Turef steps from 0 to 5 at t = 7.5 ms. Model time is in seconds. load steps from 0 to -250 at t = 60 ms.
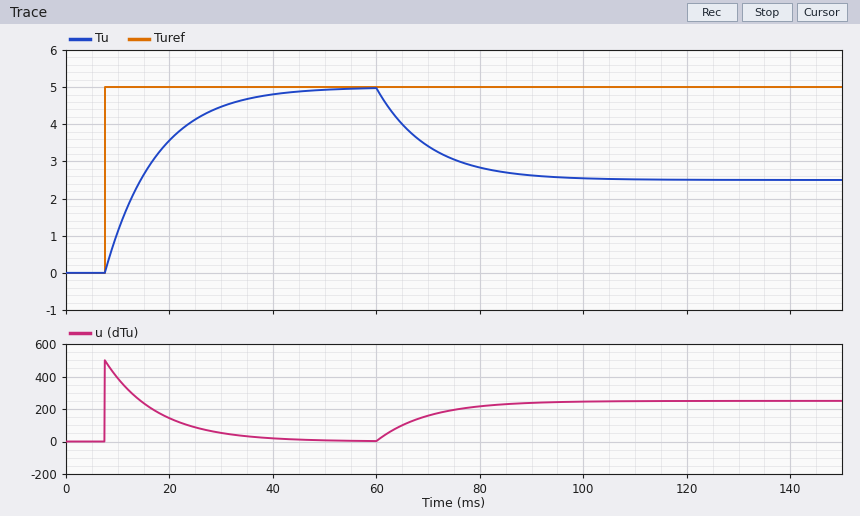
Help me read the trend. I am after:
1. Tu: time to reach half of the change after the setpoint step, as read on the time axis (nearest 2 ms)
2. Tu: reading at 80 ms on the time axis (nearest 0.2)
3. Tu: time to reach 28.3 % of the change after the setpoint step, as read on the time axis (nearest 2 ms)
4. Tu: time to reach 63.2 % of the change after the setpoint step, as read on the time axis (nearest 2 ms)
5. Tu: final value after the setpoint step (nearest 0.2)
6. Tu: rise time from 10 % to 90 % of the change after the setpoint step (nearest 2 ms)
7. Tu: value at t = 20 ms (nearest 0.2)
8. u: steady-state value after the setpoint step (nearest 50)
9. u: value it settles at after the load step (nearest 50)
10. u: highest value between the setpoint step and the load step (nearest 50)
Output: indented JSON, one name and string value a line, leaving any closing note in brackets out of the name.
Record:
{
  "Tu: time to reach half of the change after the setpoint step, as read on the time axis": "14 ms",
  "Tu: reading at 80 ms on the time axis": "2.8",
  "Tu: time to reach 28.3 % of the change after the setpoint step, as read on the time axis": "10 ms",
  "Tu: time to reach 63.2 % of the change after the setpoint step, as read on the time axis": "18 ms",
  "Tu: final value after the setpoint step": "5.0",
  "Tu: rise time from 10 % to 90 % of the change after the setpoint step": "22 ms",
  "Tu: value at t = 20 ms": "3.6",
  "u: steady-state value after the setpoint step": "0",
  "u: value it settles at after the load step": "250",
  "u: highest value between the setpoint step and the load step": "500"
}
